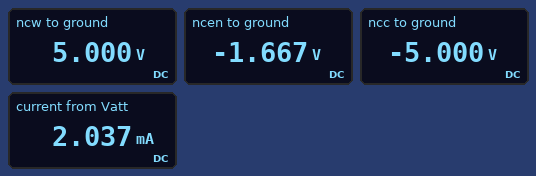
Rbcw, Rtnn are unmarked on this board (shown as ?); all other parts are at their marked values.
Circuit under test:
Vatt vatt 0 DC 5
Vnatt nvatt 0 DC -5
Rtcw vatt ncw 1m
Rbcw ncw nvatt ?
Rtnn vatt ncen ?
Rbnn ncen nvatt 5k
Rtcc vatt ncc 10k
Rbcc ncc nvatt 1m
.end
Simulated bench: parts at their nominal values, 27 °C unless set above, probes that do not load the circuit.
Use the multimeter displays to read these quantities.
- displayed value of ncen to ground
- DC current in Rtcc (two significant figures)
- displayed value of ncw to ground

-1.667 V
1.0 mA
5.000 V
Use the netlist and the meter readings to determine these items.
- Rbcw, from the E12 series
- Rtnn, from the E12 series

27 kΩ
10 kΩ
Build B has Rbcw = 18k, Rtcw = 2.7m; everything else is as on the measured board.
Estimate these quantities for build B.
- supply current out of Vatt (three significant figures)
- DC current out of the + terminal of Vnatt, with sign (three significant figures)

2.22 mA
-2.22 mA
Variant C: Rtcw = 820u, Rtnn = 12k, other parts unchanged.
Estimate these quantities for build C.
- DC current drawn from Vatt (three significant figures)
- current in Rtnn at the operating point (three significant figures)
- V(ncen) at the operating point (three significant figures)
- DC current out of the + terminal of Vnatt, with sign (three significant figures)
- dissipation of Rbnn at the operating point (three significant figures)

1.96 mA
588 µA
-2.06 V
-1.96 mA
1.73 mW
